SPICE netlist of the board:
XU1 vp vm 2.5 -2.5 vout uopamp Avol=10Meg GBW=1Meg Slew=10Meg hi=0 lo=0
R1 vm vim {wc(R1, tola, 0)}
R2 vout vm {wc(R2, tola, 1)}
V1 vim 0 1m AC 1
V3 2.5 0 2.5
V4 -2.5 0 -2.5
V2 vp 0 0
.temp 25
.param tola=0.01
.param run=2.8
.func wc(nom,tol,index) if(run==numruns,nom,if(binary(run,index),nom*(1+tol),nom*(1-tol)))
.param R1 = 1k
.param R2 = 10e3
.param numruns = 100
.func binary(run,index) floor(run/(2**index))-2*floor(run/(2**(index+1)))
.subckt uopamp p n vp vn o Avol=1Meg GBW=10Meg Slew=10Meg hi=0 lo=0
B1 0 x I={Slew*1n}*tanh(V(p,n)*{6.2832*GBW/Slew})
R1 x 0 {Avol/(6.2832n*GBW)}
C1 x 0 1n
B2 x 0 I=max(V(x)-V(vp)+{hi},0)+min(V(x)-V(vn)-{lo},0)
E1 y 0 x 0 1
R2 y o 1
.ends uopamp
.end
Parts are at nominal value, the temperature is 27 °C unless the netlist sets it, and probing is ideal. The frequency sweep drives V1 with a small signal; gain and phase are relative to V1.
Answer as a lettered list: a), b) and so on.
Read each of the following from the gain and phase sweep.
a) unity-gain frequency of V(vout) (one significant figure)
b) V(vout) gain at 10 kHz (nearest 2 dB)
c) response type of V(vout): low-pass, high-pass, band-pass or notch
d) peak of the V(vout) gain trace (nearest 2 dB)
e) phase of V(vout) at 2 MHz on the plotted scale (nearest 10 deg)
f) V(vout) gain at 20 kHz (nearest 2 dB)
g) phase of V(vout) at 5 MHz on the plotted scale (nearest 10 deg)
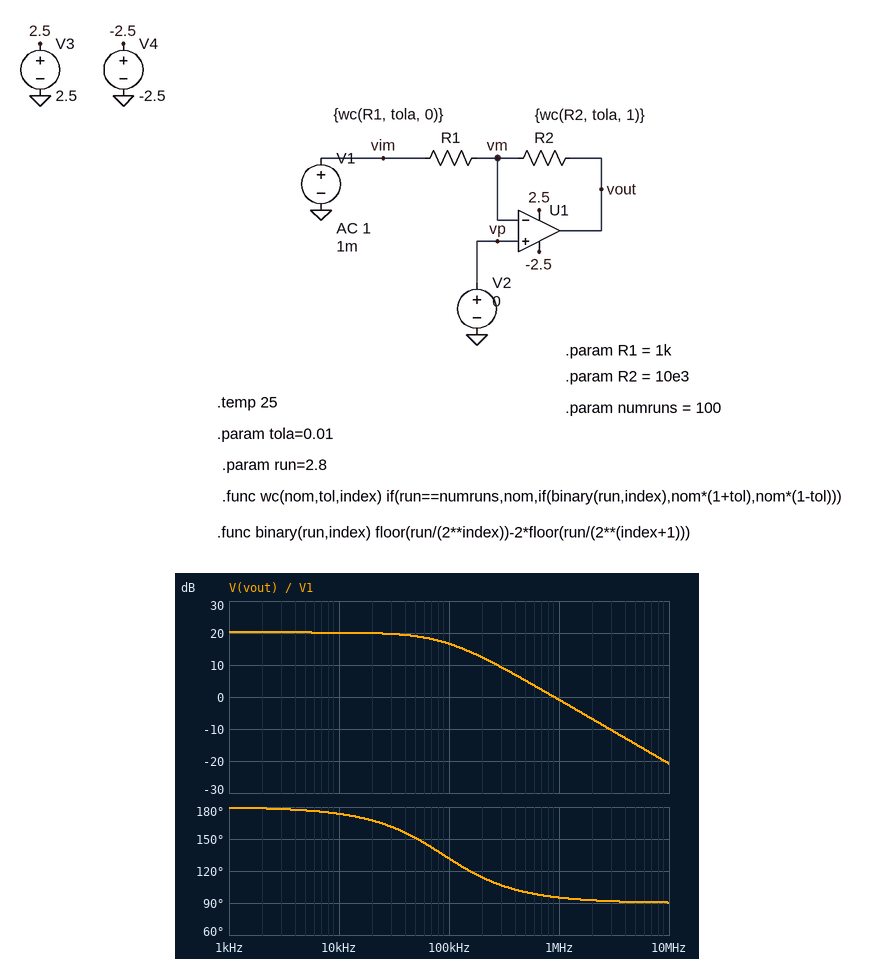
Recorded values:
a) 900 kHz
b) 20 dB
c) low-pass
d) 20 dB
e) 90 deg
f) 20 dB
g) 90 deg
